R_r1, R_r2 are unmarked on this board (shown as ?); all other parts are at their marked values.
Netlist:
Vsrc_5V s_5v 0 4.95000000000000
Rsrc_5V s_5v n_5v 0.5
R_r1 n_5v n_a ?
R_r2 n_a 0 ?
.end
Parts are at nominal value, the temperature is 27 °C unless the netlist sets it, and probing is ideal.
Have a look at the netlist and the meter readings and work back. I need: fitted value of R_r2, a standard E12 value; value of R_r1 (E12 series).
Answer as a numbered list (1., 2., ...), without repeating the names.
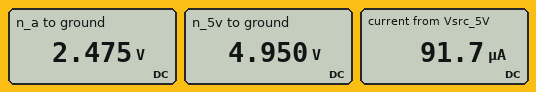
1. 27 kΩ
2. 27 kΩ
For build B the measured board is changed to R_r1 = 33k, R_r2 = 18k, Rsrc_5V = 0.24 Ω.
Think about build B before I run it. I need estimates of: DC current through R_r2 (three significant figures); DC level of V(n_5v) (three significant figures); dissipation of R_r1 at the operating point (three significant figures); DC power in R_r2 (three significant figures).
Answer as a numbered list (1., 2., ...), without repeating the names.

1. 97.1 µA
2. 4.95 V
3. 311 µW
4. 170 µW
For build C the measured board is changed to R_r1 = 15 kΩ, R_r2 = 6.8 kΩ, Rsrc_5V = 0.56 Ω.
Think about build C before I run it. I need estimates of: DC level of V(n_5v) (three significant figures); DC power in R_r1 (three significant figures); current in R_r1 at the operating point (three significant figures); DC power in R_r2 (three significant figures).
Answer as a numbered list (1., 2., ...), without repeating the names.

1. 4.95 V
2. 773 µW
3. 227 µA
4. 351 µW
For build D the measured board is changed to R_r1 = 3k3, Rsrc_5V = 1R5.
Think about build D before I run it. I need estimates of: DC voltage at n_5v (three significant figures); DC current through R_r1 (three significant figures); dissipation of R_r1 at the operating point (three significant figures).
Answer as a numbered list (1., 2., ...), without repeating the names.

1. 4.95 V
2. 163 µA
3. 88.1 µW
